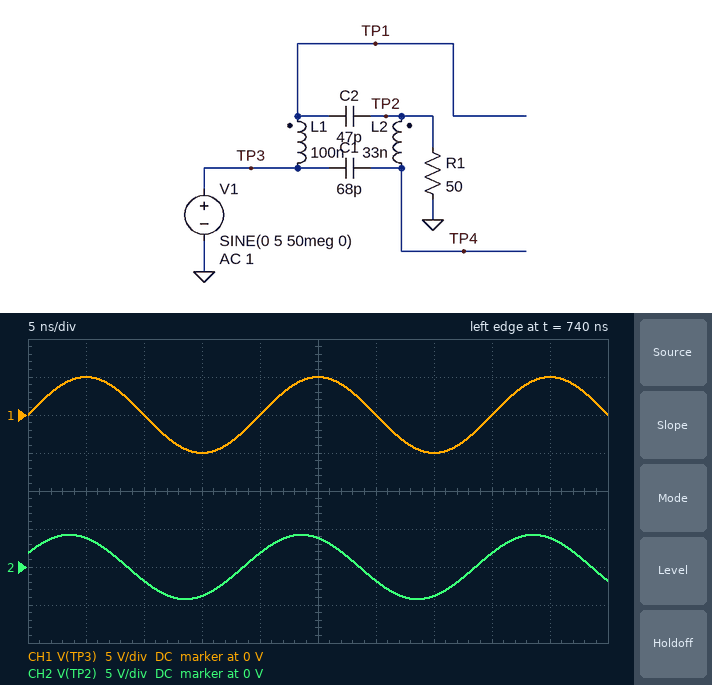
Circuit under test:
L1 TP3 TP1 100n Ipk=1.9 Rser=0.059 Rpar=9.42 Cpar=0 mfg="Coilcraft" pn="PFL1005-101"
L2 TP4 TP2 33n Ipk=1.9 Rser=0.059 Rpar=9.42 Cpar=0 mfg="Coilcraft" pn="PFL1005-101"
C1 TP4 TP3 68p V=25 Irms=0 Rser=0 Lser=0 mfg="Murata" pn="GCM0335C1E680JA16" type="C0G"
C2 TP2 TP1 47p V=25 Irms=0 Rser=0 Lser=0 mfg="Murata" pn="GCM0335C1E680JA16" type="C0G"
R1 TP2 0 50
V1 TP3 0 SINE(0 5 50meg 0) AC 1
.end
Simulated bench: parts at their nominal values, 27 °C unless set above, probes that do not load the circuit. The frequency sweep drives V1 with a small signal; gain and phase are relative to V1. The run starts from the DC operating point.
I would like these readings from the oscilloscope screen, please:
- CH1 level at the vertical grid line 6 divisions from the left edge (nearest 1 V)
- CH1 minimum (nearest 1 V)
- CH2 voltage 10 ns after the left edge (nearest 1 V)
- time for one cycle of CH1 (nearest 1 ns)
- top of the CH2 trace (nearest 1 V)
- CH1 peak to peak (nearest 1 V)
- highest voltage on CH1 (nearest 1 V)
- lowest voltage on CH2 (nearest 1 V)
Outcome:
0 V
-5 V
-2 V
20 ns
4 V
10 V
5 V
-4 V
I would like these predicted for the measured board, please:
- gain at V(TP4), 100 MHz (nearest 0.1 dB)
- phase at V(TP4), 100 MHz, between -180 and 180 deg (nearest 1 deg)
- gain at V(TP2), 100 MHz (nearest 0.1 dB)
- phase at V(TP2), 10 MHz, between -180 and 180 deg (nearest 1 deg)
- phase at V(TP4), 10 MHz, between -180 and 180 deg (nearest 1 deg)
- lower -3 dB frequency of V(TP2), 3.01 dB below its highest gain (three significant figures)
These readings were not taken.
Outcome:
-0.1 dB
15 deg
-0.9 dB
70 deg
71 deg
23.3 MHz
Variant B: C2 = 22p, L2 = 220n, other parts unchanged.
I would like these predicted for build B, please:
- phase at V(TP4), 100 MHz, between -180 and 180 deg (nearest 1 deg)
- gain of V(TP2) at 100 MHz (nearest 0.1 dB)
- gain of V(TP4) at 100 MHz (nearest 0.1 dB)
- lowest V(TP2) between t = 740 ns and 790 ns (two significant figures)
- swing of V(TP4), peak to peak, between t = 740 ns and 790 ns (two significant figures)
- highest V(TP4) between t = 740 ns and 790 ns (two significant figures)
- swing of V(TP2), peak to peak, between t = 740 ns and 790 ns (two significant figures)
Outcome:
17 deg
-1.4 dB
-0.2 dB
-3.8 V
8.7 V
4.3 V
7.6 V
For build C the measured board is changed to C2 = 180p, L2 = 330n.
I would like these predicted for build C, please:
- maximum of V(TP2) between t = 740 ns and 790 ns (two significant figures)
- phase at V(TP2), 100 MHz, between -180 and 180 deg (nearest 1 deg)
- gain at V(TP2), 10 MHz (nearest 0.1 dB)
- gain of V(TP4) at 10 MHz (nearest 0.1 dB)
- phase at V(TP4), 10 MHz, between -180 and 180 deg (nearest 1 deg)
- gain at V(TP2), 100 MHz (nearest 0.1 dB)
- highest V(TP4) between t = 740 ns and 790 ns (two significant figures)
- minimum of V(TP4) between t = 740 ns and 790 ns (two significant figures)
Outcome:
4.4 V
6 deg
-4.2 dB
-3.8 dB
51 deg
-1.0 dB
4.6 V
-4.6 V
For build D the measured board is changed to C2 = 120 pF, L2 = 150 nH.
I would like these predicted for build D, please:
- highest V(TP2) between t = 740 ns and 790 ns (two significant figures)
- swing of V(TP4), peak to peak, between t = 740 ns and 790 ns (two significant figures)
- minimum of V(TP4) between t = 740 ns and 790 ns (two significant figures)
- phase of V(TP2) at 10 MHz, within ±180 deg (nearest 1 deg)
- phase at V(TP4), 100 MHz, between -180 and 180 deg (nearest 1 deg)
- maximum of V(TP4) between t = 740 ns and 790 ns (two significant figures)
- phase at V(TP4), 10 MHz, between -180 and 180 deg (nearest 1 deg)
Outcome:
4.4 V
9.3 V
-4.7 V
58 deg
9 deg
4.7 V
60 deg
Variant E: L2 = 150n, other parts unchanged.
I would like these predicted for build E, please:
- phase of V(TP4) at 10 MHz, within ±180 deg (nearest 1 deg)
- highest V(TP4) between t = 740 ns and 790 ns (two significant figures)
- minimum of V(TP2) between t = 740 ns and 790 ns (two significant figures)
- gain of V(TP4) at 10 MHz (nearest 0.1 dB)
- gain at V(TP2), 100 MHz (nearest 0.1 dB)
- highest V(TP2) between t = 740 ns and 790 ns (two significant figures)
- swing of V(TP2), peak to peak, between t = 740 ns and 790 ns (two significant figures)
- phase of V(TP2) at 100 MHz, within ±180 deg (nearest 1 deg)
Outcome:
72 deg
4.6 V
-4.1 V
-8.8 dB
-1.0 dB
4.1 V
8.2 V
14 deg
